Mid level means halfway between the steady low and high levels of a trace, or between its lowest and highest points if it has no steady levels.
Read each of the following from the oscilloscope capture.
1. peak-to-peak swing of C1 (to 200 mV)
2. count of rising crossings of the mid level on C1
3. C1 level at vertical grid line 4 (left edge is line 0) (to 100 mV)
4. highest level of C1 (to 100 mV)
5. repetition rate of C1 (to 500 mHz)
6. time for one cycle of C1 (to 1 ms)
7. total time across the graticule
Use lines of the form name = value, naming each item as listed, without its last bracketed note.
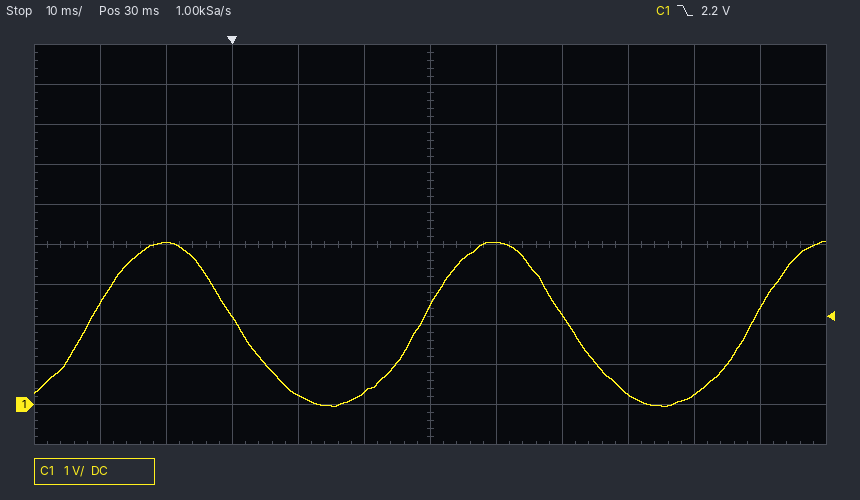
peak-to-peak swing of C1 = 4.2 V
count of rising crossings of the mid level on C1 = 3
C1 level at vertical grid line 4 (left edge is line 0) = 200 mV
highest level of C1 = 4.1 V
repetition rate of C1 = 20.0 Hz
time for one cycle of C1 = 50 ms
total time across the graticule = 120 ms
